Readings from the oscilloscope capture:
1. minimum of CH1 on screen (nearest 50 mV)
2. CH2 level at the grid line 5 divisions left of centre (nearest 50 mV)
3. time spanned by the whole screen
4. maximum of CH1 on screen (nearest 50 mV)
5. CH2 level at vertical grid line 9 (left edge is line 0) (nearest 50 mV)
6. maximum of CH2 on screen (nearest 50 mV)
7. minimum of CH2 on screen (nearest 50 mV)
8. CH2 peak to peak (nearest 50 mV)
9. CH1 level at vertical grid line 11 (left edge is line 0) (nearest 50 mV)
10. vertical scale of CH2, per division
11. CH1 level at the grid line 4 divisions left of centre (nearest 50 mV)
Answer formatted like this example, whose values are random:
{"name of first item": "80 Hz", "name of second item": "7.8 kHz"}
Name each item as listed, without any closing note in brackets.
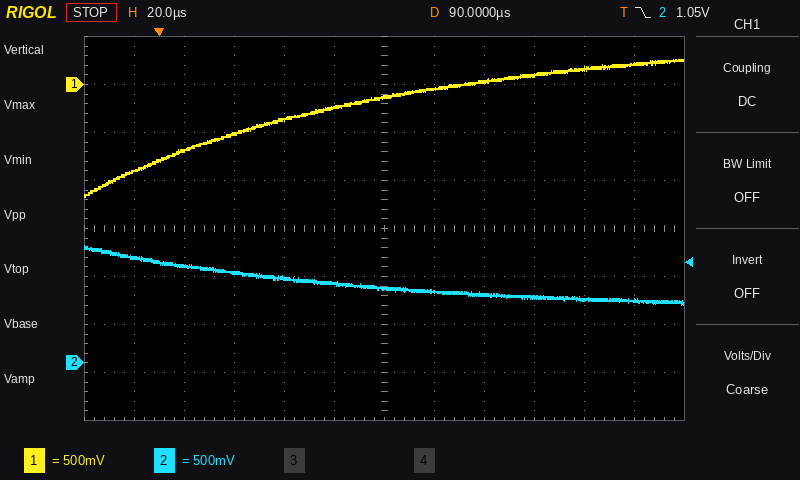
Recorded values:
{"minimum of CH1 on screen": "-1.15 V", "CH2 level at the grid line 5 divisions left of centre": "1.10 V", "time spanned by the whole screen": "240 µs", "maximum of CH1 on screen": "250 mV", "CH2 level at vertical grid line 9 (left edge is line 0)": "700 mV", "maximum of CH2 on screen": "1.20 V", "minimum of CH2 on screen": "600 mV", "CH2 peak to peak": "600 mV", "CH1 level at vertical grid line 11 (left edge is line 0)": "200 mV", "vertical scale of CH2, per division": "500 mV", "CH1 level at the grid line 4 divisions left of centre": "-700 mV"}
